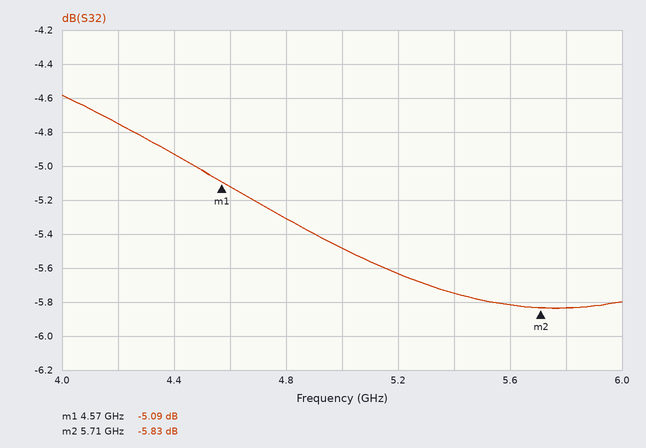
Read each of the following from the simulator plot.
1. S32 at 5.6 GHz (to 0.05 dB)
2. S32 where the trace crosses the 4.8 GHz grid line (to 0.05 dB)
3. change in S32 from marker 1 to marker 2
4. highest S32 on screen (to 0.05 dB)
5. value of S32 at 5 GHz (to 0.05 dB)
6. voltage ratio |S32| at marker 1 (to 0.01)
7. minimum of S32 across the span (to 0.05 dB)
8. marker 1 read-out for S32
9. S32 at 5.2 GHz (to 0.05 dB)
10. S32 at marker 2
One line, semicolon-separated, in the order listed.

-5.80 dB; -5.30 dB; -0.74 dB; -4.60 dB; -5.50 dB; 0.56; -5.85 dB; -5.09 dB; -5.65 dB; -5.83 dB
